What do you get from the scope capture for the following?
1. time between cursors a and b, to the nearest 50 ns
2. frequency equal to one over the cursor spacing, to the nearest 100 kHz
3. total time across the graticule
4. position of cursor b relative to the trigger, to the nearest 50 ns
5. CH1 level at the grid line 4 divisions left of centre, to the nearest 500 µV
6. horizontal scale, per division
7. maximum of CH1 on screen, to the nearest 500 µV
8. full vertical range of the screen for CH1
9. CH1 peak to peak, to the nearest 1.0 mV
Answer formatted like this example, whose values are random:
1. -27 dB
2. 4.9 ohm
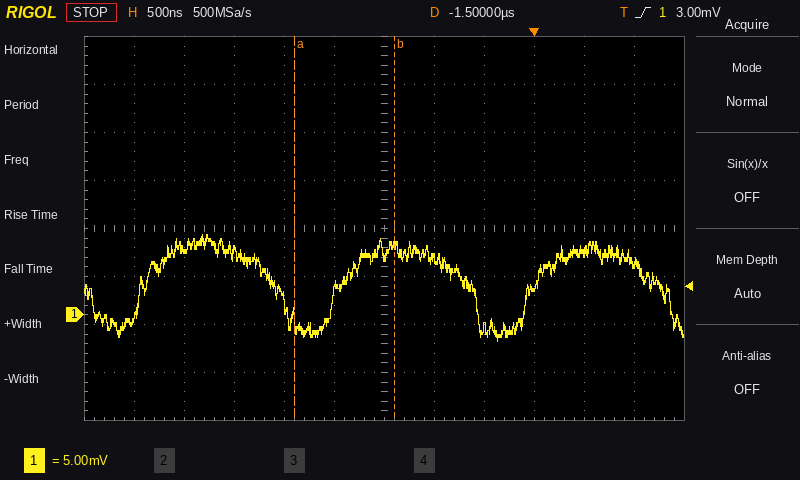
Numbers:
1. 1.00 µs
2. 1.0 MHz
3. 6 µs
4. -1.40 µs
5. 7.0 mV
6. 500 ns
7. 8.5 mV
8. 40 mV
9. 11.0 mV
